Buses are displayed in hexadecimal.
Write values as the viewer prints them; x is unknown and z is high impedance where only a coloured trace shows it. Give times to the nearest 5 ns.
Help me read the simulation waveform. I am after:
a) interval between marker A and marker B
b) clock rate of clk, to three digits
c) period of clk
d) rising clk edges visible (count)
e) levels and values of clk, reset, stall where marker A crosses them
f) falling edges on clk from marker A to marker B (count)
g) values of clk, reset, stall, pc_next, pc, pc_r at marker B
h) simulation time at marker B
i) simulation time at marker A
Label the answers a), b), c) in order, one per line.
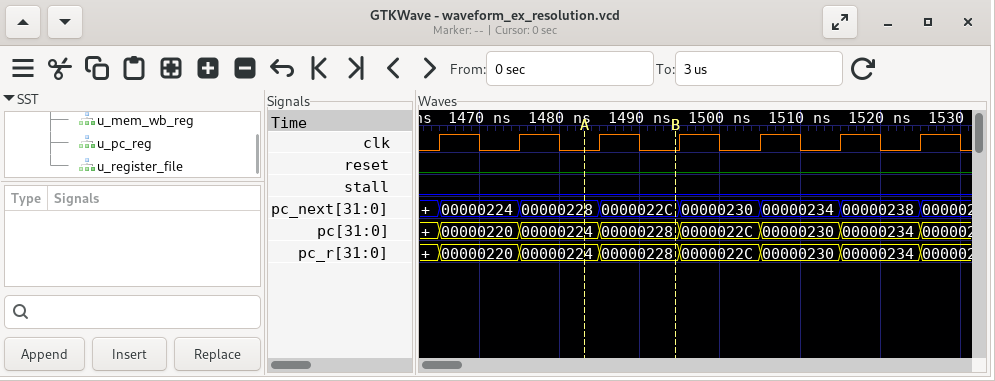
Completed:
a) 10 ns
b) 100 MHz
c) 10 ns
d) 7
e) clk=0, reset=0, stall=0
f) 1
g) clk=0, reset=0, stall=0, pc_next=0000022C, pc=00000228, pc_r=00000228
h) 1495 ns
i) 1485 ns
